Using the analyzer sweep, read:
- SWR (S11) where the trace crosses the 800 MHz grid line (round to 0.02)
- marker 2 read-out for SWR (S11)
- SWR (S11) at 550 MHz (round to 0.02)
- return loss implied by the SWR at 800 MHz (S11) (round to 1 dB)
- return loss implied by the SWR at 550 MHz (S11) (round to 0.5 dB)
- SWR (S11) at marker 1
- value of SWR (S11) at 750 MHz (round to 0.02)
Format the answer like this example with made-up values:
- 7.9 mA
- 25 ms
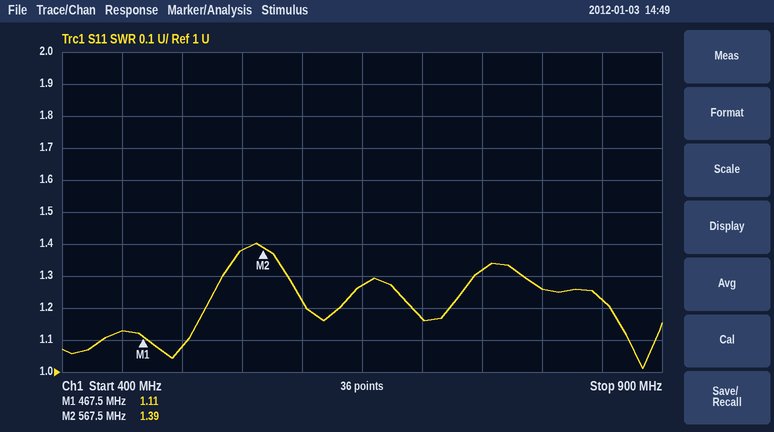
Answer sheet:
- 1.26
- 1.39
- 1.38
- 19 dB
- 16.0 dB
- 1.11
- 1.32
